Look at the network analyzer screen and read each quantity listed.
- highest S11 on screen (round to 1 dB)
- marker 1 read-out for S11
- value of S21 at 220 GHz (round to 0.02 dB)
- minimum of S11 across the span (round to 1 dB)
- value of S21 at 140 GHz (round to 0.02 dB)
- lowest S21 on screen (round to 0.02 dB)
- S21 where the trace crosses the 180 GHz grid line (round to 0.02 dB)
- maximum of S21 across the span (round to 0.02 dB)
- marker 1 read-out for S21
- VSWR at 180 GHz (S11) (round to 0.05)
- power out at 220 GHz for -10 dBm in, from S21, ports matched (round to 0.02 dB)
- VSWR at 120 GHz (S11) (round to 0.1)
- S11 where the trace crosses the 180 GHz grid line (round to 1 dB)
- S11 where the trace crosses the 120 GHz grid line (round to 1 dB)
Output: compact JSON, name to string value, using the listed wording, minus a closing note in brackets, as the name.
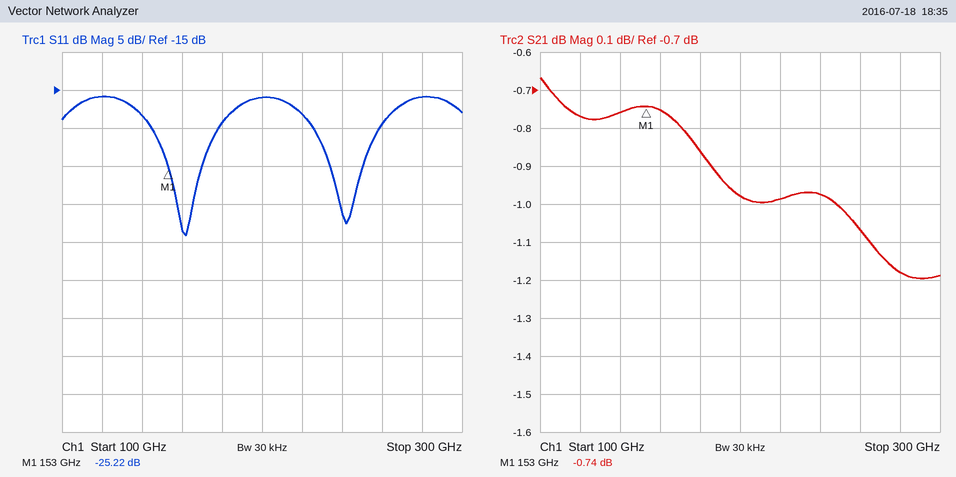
{"highest S11 on screen": "-16 dB", "marker 1 read-out for S11": "-25.22 dB", "value of S21 at 220 GHz": "-0.98 dB", "minimum of S11 across the span": "-34 dB", "value of S21 at 140 GHz": "-0.76 dB", "lowest S21 on screen": "-1.20 dB", "S21 where the trace crosses the 180 GHz grid line": "-0.86 dB", "maximum of S21 across the span": "-0.66 dB", "marker 1 read-out for S21": "-0.74 dB", "VSWR at 180 GHz (S11)": "1.25", "power out at 220 GHz for -10 dBm in, from S21, ports matched": "-10.98 dBm", "VSWR at 120 GHz (S11)": "1.4", "S11 where the trace crosses the 180 GHz grid line": "-19 dB", "S11 where the trace crosses the 120 GHz grid line": "-16 dB"}
